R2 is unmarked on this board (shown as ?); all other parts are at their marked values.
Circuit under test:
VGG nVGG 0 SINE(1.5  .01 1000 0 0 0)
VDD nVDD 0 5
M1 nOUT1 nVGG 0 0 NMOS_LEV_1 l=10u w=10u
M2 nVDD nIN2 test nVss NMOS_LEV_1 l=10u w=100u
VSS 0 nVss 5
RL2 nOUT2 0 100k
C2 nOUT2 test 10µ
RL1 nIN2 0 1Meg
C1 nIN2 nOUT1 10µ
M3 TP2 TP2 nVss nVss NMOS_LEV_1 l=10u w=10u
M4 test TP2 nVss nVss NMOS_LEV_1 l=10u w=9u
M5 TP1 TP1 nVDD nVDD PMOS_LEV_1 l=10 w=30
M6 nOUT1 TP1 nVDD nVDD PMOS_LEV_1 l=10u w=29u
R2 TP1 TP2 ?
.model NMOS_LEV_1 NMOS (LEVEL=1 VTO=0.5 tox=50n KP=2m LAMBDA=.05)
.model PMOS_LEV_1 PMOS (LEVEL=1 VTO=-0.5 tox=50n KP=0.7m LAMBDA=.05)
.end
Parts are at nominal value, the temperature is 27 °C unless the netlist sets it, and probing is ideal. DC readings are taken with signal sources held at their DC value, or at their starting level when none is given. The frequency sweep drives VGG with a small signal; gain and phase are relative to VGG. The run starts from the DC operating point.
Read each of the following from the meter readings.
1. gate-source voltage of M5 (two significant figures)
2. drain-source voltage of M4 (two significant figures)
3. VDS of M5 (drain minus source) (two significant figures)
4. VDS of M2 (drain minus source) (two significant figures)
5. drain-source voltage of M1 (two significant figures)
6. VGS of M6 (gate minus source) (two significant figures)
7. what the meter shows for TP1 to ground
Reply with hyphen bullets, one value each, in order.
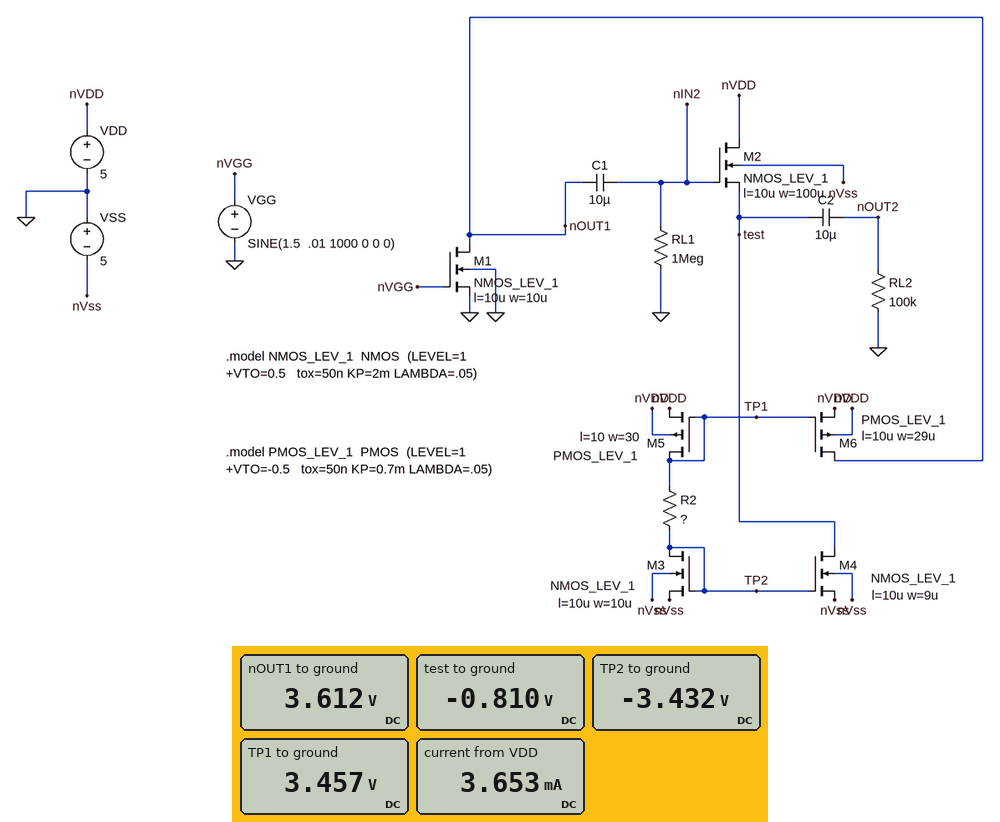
- -1.5 V
- 4.2 V
- -1.5 V
- 5.8 V
- 3.6 V
- -1.5 V
- 3.457 V
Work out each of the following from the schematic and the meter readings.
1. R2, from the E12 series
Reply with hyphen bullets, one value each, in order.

- 5.6 kΩ
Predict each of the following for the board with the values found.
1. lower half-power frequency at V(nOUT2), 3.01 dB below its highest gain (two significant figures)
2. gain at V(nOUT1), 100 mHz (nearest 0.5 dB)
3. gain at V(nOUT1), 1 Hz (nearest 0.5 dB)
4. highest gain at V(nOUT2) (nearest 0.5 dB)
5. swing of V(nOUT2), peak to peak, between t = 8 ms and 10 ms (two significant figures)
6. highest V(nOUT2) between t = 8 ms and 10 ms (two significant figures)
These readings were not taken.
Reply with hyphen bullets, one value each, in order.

- 160 mHz
- 27.0 dB
- 27.0 dB
- 27.0 dB
- 440 mV
- 220 mV
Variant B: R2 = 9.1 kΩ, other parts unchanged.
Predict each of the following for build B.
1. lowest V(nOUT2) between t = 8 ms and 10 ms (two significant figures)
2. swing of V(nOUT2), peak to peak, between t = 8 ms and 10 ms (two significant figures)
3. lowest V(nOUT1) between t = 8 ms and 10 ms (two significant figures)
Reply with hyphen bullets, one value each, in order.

- -14 mV
- 30 mV
- 610 mV
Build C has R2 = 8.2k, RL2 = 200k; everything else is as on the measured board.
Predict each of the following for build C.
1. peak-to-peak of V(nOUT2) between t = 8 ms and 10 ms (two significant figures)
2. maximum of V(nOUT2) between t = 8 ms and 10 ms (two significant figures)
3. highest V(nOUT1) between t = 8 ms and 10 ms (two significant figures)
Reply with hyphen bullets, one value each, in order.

- 48 mV
- 26 mV
- 760 mV
